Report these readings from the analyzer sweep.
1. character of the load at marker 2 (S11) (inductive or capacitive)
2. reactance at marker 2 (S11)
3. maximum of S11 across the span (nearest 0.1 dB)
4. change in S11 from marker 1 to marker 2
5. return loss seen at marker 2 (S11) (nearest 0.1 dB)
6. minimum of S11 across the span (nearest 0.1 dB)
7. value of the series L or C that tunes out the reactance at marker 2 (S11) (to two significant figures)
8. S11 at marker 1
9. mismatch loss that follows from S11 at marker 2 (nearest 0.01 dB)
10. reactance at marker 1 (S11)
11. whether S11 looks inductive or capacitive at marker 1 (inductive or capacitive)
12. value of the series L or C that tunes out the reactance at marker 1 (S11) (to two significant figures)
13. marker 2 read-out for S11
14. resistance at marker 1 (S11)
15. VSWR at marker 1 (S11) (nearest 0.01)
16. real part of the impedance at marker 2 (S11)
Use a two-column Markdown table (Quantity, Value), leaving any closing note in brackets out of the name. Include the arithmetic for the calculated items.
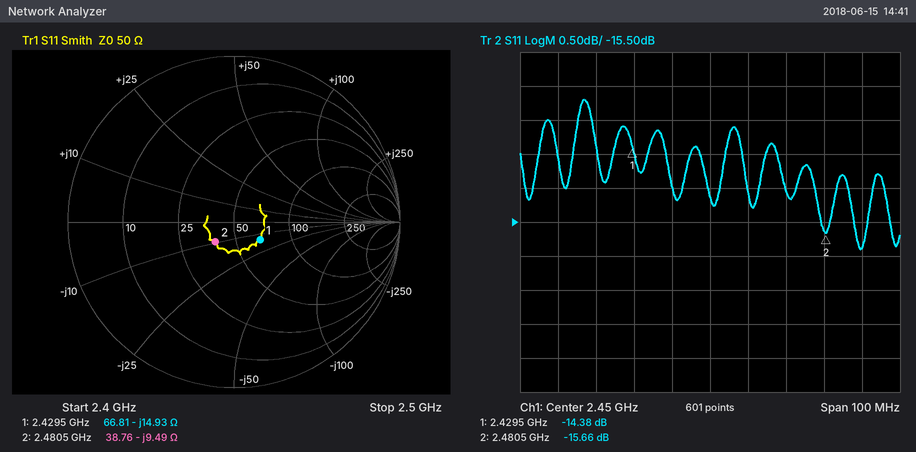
| Quantity | Value |
|---|---|
| character of the load at marker 2 (S11) | capacitive |
| reactance at marker 2 | -9.49 Ω |
| maximum of S11 across the span | -13.7 dB |
| change in S11 from marker 1 to marker 2 | -15.66 − (-14.38) = -1.28 dB |
| return loss seen at marker 2 (S11) | 15.7 dB |
| minimum of S11 across the span | -15.9 dB |
| value of the series L or C that tunes out the reactance at marker 2 (S11) | L = 9.49 Ω/(2π × 2.4805 GHz) ≈ 609 pH, so 610 pH to two significant figures |
| S11 at marker 1 | -14.38 dB |
| mismatch loss that follows from S11 at marker 2 | −10 log10(1 − 10^(-15.66/10)) ≈ 0.12 dB |
| reactance at marker 1 | -14.93 Ω |
| whether S11 looks inductive or capacitive at marker 1 | capacitive |
| value of the series L or C that tunes out the reactance at marker 1 (S11) | L = 14.93 Ω/(2π × 2.4295 GHz) ≈ 978 pH, so 980 pH to two significant figures |
| marker 2 read-out for S11 | -15.66 dB |
| resistance at marker 1 | 66.81 Ω |
| VSWR at marker 1 (S11) | 1.47 |
| real part of the impedance at marker 2 | 38.76 Ω |
